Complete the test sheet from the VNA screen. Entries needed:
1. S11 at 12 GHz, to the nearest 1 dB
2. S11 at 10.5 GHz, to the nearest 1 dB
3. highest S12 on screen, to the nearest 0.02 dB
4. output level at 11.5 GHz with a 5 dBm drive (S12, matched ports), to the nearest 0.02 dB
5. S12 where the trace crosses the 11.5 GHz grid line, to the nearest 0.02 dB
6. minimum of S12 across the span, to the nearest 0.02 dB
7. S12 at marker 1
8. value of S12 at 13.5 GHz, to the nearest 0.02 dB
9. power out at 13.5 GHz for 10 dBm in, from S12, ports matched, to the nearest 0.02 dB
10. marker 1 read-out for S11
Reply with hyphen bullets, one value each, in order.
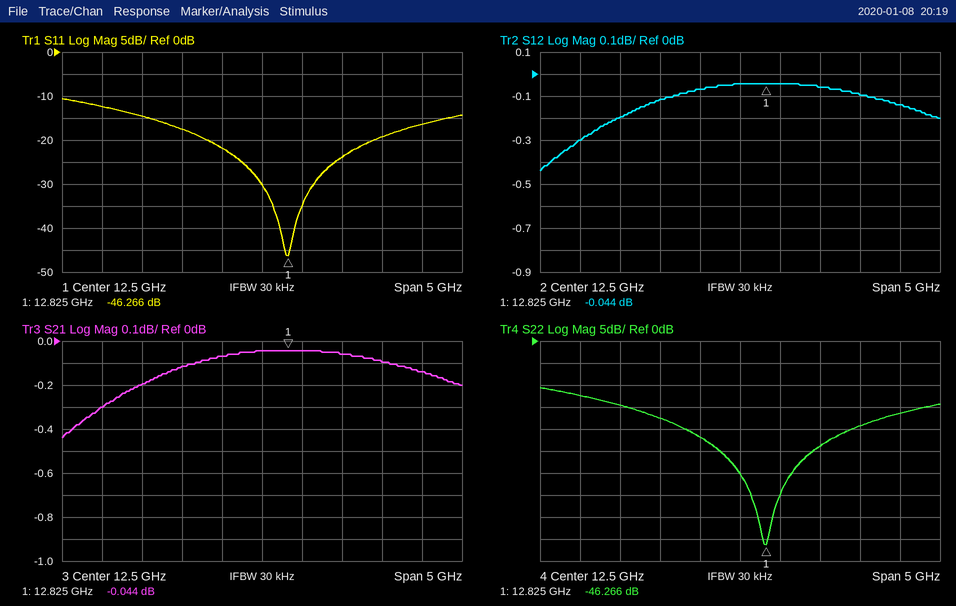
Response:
- -22 dB
- -12 dB
- -0.04 dB
- 4.88 dBm
- -0.12 dB
- -0.44 dB
- -0.044 dB
- -0.06 dB
- 9.94 dBm
- -46.266 dB
